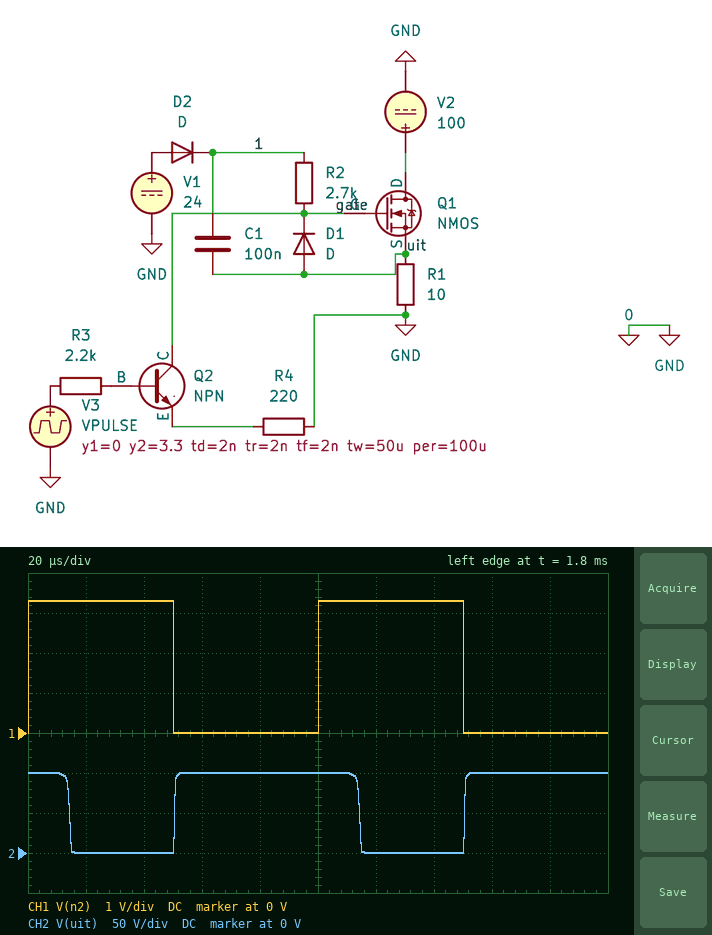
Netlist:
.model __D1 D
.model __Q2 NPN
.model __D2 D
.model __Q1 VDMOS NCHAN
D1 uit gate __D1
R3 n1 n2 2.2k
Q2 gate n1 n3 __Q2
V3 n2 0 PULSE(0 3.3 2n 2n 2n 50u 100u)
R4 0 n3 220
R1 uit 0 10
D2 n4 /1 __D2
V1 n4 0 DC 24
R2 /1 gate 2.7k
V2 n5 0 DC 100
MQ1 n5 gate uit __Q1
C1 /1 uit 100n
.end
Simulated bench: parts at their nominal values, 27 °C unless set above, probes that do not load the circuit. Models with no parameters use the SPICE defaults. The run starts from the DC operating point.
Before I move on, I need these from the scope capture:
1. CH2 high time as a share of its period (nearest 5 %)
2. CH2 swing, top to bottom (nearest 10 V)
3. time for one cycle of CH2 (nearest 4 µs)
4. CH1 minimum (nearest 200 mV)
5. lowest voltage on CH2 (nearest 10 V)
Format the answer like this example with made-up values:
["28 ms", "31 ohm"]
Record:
["65 %", "100 V", "100 µs", "0 V", "0 V"]
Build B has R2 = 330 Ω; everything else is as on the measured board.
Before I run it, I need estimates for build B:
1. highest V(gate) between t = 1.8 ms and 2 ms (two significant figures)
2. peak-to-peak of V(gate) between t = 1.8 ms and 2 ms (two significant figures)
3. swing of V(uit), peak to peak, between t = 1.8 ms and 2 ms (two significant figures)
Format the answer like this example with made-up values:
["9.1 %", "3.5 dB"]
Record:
["110 V", "87 V", "84 V"]
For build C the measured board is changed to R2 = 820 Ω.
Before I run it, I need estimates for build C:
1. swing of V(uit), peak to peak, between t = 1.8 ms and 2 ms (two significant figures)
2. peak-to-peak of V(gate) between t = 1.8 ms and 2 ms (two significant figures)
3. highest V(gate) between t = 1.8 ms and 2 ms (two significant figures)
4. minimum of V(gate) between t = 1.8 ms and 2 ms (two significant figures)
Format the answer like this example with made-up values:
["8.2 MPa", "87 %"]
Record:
["89 V", "97 V", "110 V", "14 V"]
